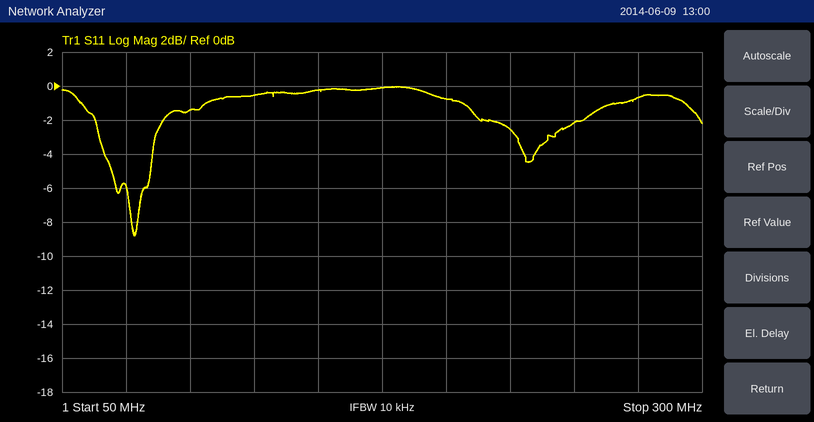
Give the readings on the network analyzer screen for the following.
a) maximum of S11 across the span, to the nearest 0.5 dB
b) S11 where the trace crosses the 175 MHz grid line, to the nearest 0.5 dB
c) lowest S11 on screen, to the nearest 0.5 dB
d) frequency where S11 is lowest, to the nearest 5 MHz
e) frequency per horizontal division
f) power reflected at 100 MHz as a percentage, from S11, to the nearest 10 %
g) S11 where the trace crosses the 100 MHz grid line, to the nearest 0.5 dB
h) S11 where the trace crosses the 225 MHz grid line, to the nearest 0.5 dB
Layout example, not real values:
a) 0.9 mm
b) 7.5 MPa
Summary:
a) 0.0 dB
b) 0.0 dB
c) -9.0 dB
d) 80 MHz
e) 25 MHz
f) 70 %
g) -1.5 dB
h) -2.5 dB
